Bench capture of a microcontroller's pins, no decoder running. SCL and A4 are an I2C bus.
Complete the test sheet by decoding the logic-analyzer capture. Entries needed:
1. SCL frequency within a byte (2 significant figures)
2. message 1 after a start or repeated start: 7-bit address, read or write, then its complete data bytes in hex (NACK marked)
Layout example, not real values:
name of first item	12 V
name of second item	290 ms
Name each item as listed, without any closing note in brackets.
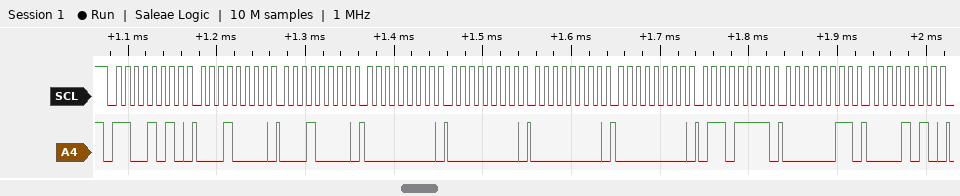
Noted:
SCL frequency within a byte	100 kHz
message 1 after a start or repeated start: 7-bit address, read or write, then its complete data bytes in hex	0x65 write: 10 10 00 00 00 00 6F 03 0A
